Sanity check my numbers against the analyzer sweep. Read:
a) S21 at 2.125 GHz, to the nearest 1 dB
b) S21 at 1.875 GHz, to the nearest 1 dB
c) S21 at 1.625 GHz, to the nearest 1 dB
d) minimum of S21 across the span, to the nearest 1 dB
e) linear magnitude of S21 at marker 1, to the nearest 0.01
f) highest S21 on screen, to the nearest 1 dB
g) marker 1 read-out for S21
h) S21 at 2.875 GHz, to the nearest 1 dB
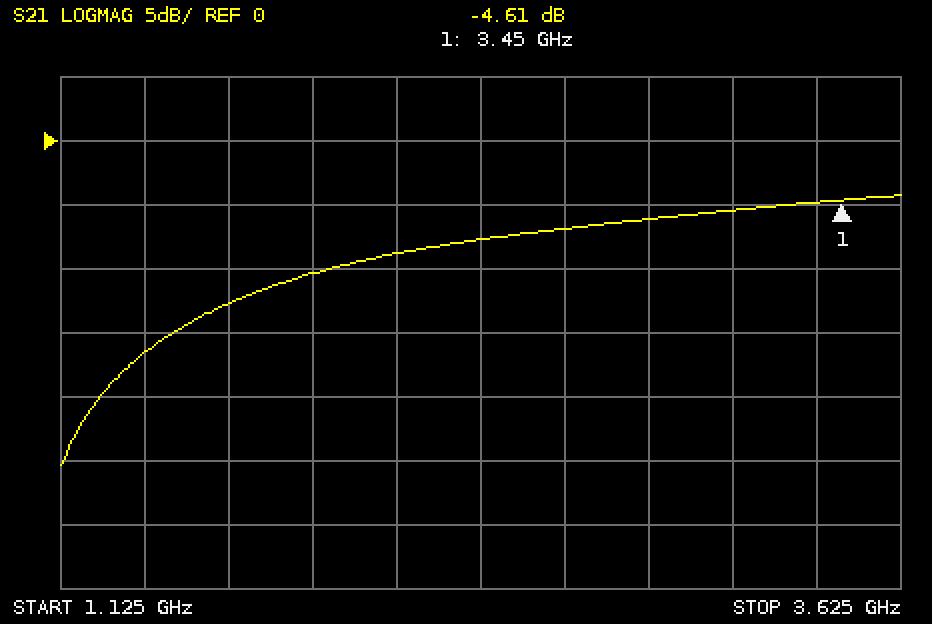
-9 dB
-10 dB
-13 dB
-25 dB
0.59
-4 dB
-4.61 dB
-6 dB
